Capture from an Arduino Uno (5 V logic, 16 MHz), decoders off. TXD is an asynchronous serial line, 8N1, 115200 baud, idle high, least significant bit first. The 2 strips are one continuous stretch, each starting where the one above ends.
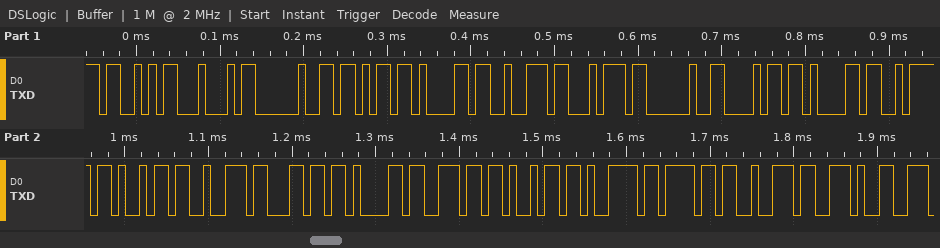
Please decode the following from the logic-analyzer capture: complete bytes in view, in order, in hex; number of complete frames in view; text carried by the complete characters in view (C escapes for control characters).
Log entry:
53 44 20 6B 61 72 74 20 68 61 7A 69 72 6C 61 6E 69 79 6F 72 2E
21
"SD kart hazirlaniyor."
